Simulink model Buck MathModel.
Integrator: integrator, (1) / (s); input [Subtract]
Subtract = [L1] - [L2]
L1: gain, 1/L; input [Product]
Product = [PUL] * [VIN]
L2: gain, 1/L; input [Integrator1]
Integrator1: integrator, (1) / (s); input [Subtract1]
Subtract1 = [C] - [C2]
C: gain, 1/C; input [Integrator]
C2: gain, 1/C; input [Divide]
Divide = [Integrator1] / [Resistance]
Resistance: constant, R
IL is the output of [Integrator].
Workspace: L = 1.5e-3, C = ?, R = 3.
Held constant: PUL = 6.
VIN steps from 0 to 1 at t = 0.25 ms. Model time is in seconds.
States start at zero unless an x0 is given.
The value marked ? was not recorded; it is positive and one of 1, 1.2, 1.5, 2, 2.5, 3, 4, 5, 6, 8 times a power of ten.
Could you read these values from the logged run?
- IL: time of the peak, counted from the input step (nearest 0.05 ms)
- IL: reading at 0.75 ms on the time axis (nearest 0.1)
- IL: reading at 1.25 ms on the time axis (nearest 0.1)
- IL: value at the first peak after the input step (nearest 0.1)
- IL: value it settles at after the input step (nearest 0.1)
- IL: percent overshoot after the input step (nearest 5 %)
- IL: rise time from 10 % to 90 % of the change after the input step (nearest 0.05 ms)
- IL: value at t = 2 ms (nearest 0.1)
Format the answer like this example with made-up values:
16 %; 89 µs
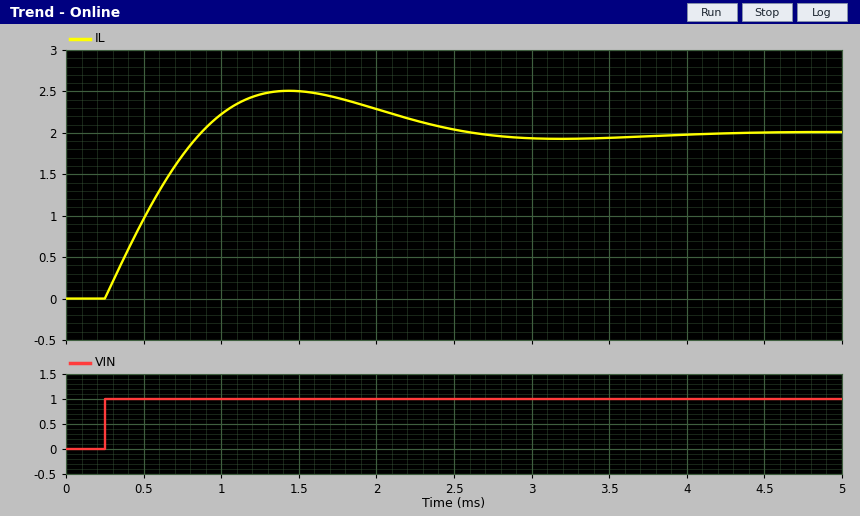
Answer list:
1.20 ms; 1.7; 2.5; 2.5; 2.0; 25 %; 0.50 ms; 2.3
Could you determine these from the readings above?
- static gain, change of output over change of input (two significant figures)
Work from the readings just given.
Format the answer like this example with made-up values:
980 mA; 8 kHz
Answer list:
2.0
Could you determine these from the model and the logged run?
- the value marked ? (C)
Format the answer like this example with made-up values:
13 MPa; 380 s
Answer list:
0.00015
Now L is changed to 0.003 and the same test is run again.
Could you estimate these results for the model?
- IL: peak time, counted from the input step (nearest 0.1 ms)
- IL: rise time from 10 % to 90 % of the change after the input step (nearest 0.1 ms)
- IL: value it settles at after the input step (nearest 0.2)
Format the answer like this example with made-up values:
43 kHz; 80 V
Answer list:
2.4 ms; 1.2 ms; 2.0
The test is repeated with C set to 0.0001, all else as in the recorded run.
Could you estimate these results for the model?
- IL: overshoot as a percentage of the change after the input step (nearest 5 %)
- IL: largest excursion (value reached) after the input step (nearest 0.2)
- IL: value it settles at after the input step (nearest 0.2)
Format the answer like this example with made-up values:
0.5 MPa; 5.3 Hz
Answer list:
10 %; 2.2; 2.0
